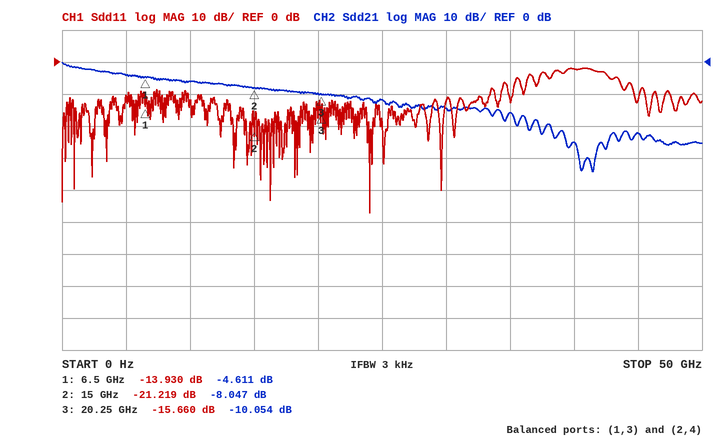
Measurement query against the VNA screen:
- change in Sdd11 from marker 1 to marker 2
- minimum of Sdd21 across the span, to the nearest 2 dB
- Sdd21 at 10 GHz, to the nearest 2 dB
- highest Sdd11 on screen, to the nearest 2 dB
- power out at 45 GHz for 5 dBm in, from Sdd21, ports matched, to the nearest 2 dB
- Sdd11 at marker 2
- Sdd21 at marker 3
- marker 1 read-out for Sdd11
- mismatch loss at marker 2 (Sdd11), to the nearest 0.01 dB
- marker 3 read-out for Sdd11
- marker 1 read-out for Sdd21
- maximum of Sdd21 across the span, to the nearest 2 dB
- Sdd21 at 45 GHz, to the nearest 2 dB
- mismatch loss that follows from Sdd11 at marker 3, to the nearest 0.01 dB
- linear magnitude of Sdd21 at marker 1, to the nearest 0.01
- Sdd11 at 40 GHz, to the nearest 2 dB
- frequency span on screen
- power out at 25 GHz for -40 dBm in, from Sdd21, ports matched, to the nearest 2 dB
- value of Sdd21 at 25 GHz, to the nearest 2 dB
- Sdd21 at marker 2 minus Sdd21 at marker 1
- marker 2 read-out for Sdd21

-7.289 dB
-34 dB
-6 dB
-2 dB
-18 dBm
-21.219 dB
-10.054 dB
-13.930 dB
0.03 dB
-15.660 dB
-4.611 dB
0 dB
-22 dB
0.12 dB
0.59
-2 dB
50 GHz
-52 dBm
-12 dB
-3.436 dB
-8.047 dB
